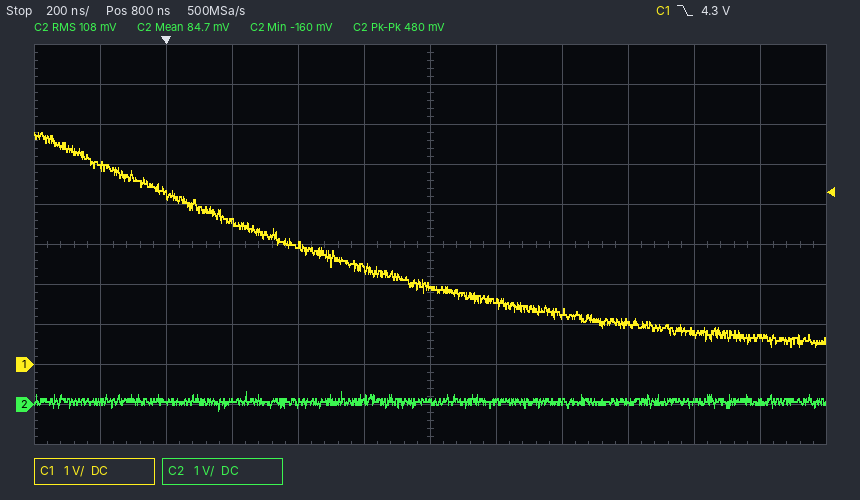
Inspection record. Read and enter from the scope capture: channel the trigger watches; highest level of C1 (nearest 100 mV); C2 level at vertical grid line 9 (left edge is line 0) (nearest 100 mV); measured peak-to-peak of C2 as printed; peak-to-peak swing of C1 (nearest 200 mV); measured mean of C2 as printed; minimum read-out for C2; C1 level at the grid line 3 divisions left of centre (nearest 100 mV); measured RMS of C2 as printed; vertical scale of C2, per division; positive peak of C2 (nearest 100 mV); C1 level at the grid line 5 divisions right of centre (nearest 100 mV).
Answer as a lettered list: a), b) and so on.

a) C1
b) 5.8 V
c) 100 mV
d) 480 mV
e) 5.4 V
f) 84.7 mV
g) -160 mV
h) 3.6 V
i) 108 mV
j) 1 V
k) 300 mV
l) 700 mV
